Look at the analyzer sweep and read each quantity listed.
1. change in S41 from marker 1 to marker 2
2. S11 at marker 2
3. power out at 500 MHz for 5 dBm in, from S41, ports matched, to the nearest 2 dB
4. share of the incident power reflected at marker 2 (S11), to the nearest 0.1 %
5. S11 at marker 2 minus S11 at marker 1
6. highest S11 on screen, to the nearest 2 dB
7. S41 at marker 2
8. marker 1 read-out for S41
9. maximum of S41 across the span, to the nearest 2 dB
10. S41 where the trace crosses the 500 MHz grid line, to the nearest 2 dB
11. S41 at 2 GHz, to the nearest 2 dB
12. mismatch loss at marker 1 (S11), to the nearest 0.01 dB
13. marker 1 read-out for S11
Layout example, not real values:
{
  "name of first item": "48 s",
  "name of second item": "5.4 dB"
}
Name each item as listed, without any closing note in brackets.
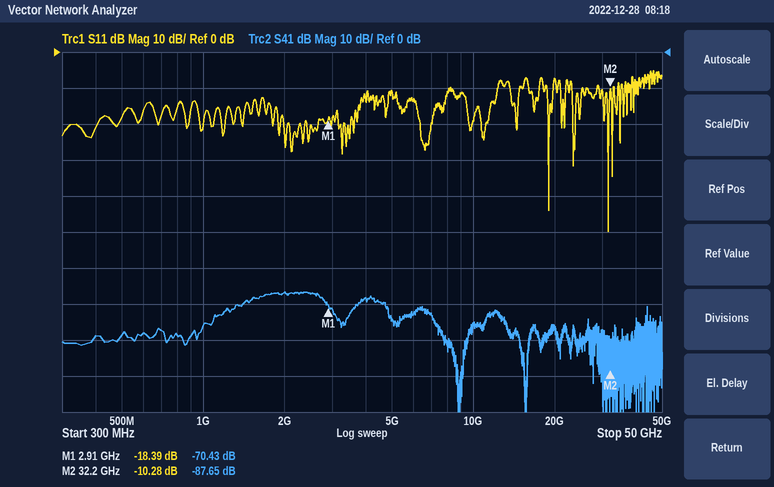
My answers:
{
  "change in S41 from marker 1 to marker 2": "-17.22 dB",
  "S11 at marker 2": "-10.28 dB",
  "power out at 500 MHz for 5 dBm in, from S41, ports matched, to the nearest 2 dB": "-74 dBm",
  "share of the incident power reflected at marker 2 (S11), to the nearest 0.1 %": "9.4 %",
  "S11 at marker 2 minus S11 at marker 1": "8.11 dB",
  "highest S11 on screen, to the nearest 2 dB": "-6 dB",
  "S41 at marker 2": "-87.65 dB",
  "marker 1 read-out for S41": "-70.43 dB",
  "maximum of S41 across the span, to the nearest 2 dB": "-66 dB",
  "S41 where the trace crosses the 500 MHz grid line, to the nearest 2 dB": "-78 dB",
  "S41 at 2 GHz, to the nearest 2 dB": "-66 dB",
  "mismatch loss at marker 1 (S11), to the nearest 0.01 dB": "0.06 dB",
  "marker 1 read-out for S11": "-18.39 dB"
}
